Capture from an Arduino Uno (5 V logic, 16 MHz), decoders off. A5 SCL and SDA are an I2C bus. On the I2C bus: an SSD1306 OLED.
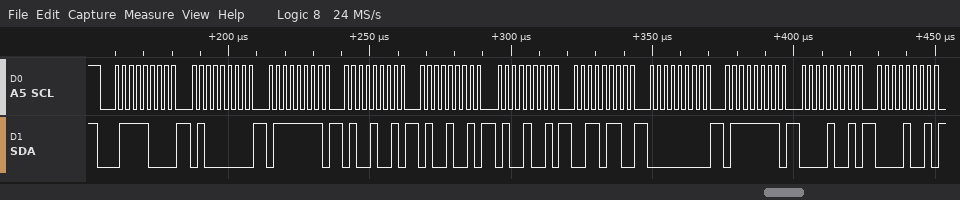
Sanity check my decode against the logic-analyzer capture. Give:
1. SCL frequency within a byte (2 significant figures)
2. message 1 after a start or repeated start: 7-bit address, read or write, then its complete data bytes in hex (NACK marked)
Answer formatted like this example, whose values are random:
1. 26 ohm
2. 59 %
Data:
1. 400 kHz
2. 0x3C write: 40 7F 49 49 49 36 00 7F 09 09
